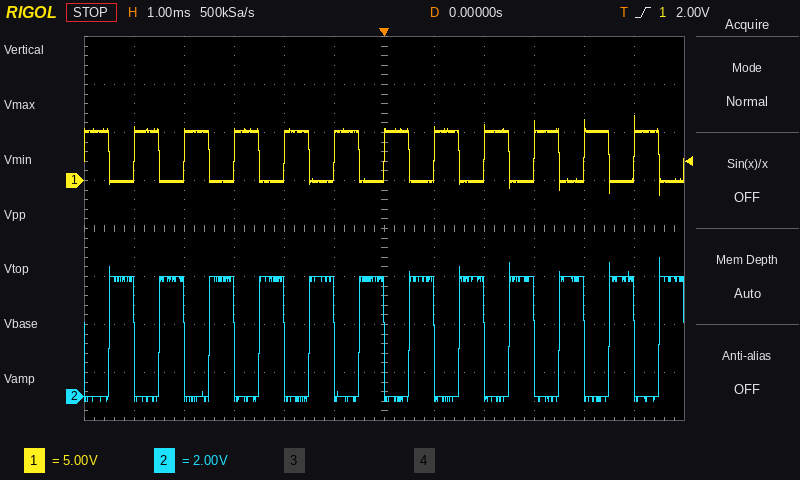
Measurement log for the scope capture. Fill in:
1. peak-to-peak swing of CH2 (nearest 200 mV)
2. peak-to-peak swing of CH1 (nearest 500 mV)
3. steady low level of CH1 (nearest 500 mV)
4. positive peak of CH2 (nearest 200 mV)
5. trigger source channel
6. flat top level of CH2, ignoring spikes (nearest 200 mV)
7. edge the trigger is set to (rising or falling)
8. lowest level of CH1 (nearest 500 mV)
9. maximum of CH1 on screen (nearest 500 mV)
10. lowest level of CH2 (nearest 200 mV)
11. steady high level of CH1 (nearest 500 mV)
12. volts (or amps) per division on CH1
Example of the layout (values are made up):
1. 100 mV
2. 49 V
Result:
1. 6.0 V
2. 8.5 V
3. 0.0 V
4. 5.8 V
5. CH1
6. 5.0 V
7. rising
8. -1.5 V
9. 7.0 V
10. -200 mV
11. 5.0 V
12. 5 V
